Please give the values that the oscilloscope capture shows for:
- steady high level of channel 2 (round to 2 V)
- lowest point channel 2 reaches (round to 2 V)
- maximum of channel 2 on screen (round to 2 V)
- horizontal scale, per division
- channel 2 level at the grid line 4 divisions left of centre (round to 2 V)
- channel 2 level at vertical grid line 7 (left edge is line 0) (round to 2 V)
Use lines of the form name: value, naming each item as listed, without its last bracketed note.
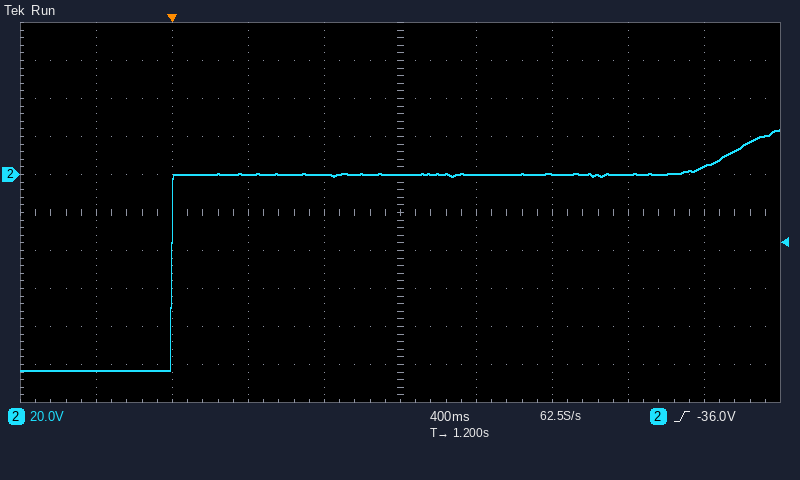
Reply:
steady high level of channel 2: 0 V
lowest point channel 2 reaches: -104 V
maximum of channel 2 on screen: 24 V
horizontal scale, per division: 400 ms
channel 2 level at the grid line 4 divisions left of centre: -104 V
channel 2 level at vertical grid line 7 (left edge is line 0): 0 V
